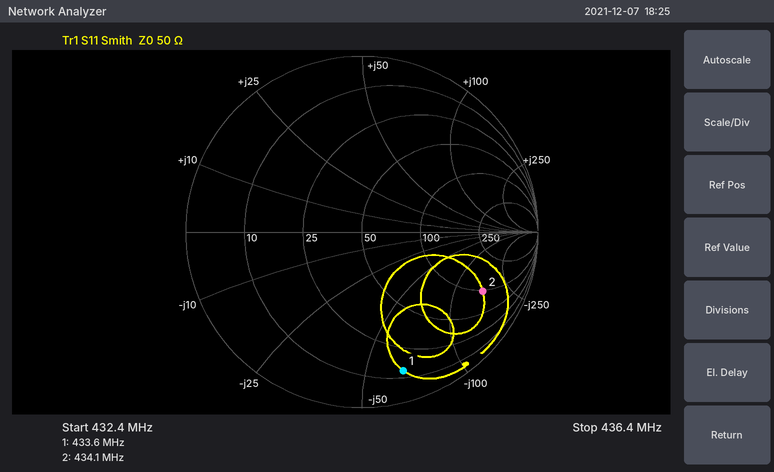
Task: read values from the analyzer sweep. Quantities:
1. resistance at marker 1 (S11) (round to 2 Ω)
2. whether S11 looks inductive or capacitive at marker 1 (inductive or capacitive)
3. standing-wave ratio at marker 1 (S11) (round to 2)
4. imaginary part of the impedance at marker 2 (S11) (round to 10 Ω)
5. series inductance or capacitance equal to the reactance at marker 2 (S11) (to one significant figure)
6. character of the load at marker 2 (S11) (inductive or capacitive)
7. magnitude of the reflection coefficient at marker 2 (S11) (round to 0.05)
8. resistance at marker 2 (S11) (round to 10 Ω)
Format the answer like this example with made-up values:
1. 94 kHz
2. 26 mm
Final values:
1. 14 Ω
2. capacitive
3. 10
4. -160 Ω
5. 2 pF
6. capacitive
7. 0.75
8. 100 Ω
